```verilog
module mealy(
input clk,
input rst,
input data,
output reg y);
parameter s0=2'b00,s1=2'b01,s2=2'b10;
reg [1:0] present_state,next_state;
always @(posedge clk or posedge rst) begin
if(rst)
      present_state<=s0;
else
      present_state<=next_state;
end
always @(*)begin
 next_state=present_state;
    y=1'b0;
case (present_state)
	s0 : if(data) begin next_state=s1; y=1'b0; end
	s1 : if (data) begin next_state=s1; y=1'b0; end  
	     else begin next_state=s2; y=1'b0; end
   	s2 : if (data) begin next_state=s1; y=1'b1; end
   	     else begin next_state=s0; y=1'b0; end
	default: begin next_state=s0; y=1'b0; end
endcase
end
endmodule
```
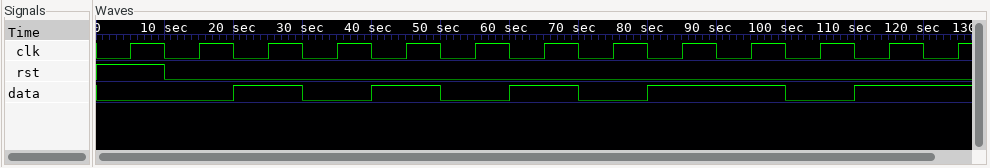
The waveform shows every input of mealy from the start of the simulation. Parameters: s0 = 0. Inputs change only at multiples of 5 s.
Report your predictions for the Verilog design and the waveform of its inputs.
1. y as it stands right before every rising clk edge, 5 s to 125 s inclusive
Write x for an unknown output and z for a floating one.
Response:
0 0 0 0 1 0 1 0 1 0 0 1 0
